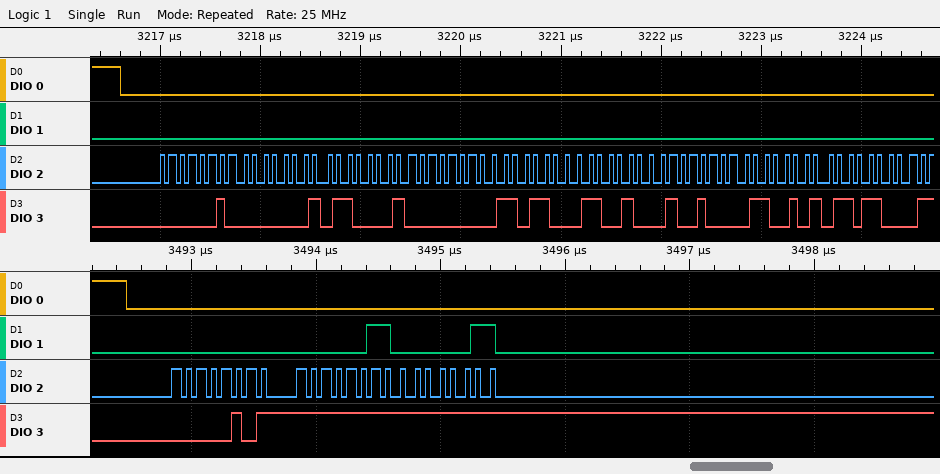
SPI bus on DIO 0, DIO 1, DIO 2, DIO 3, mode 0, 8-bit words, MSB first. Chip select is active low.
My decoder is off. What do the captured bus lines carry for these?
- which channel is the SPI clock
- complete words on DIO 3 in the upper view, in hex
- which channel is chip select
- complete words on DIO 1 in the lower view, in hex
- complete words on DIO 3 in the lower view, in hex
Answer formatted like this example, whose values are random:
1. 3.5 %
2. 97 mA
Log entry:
1. DIO 2
2. 02, 01, 61, 00, 6C, 64, 48, 65, 6C
3. DIO 0
4. 00, 03, 03
5. 05, FF, FF
